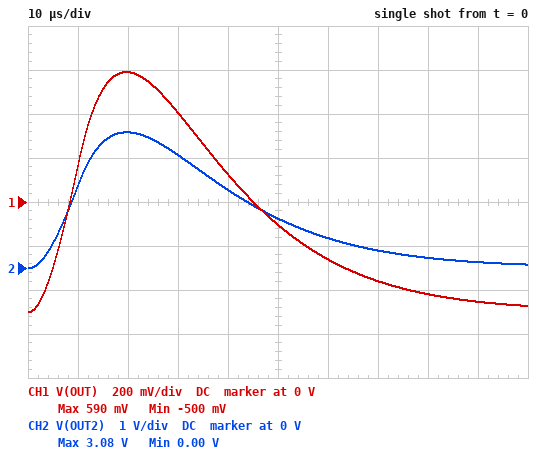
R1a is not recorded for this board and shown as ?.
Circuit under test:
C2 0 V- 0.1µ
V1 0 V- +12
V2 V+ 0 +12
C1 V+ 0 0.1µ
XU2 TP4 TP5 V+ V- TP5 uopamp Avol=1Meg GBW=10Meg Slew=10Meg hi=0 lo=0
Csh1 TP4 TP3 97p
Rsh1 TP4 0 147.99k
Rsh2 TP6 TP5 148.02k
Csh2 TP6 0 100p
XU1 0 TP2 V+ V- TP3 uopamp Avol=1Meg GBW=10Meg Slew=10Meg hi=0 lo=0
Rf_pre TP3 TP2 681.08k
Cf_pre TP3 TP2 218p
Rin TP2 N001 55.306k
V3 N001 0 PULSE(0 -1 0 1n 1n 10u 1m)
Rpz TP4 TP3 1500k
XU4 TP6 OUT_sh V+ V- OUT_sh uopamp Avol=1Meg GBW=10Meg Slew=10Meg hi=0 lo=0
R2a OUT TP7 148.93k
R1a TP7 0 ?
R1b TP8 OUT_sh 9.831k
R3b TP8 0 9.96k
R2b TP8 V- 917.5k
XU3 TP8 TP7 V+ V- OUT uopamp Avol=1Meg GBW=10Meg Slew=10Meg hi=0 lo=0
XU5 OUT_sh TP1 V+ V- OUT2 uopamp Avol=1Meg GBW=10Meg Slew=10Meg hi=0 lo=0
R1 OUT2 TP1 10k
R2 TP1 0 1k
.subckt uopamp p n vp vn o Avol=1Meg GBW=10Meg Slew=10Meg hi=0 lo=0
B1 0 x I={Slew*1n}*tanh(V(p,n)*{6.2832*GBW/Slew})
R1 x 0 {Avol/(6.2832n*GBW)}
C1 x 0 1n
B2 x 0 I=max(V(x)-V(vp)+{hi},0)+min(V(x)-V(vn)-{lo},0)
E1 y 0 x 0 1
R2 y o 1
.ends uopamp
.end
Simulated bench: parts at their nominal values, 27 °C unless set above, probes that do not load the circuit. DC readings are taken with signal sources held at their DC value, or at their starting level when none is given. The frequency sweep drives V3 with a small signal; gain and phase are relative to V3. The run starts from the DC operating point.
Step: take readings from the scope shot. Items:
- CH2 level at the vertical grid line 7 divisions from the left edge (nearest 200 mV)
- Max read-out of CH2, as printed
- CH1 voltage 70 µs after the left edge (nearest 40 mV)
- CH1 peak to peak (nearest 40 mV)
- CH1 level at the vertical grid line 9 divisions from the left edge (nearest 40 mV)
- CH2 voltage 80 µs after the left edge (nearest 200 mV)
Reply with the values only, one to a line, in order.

400 mV
3.08 V
-360 mV
1.08 V
-440 mV
200 mV
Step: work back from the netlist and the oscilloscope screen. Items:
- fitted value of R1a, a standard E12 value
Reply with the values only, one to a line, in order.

22 kΩ
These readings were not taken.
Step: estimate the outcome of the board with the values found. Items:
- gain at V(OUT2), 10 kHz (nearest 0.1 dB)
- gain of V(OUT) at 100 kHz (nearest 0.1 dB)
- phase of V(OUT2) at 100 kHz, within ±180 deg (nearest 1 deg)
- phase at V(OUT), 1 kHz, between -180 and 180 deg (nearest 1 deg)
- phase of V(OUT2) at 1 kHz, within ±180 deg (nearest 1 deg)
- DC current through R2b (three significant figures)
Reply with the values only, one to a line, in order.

16.6 dB
-25.3 dB
5 deg
169 deg
169 deg
13.0 µA
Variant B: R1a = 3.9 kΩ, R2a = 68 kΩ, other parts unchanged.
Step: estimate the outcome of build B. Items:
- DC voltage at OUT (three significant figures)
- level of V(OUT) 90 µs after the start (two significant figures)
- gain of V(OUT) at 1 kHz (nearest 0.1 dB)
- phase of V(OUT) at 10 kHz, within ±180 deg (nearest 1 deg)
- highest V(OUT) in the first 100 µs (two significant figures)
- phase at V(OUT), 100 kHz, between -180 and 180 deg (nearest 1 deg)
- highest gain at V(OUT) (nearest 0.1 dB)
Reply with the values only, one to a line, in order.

-1.19 V
-1.1 V
20.0 dB
96 deg
1.4 V
1 deg
20.2 dB
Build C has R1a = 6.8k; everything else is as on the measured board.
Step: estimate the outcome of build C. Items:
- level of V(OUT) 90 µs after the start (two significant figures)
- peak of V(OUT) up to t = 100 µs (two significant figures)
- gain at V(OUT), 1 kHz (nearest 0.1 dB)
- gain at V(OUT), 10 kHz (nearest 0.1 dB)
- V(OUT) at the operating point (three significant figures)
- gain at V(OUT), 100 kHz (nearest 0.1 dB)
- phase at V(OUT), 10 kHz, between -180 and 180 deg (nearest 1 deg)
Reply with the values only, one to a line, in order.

-1.3 V
1.7 V
21.9 dB
16.9 dB
-1.47 V
-16.1 dB
96 deg
